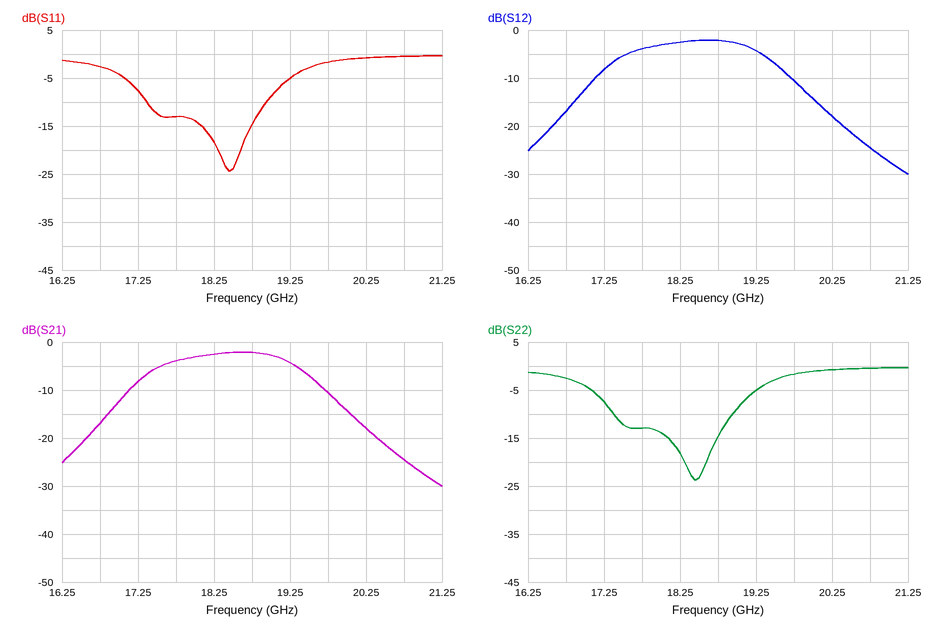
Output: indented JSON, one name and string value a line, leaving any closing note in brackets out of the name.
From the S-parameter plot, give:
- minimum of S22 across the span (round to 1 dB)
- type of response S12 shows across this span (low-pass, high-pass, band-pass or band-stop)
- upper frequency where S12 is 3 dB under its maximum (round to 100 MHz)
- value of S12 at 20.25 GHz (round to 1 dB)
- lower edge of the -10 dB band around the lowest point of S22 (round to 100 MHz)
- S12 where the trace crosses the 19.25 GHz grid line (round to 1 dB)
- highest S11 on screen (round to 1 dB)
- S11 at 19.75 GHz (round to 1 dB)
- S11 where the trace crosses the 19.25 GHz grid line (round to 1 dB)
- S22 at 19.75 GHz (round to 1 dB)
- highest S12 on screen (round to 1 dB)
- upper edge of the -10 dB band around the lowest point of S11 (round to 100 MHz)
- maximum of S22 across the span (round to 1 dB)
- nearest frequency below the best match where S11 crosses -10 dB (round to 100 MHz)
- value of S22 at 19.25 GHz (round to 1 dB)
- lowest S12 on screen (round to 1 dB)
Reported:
{
  "minimum of S22 across the span": "-24 dB",
  "type of response S12 shows across this span": "band-pass",
  "upper frequency where S12 is 3 dB under its maximum": "19.3 GHz",
  "value of S12 at 20.25 GHz": "-18 dB",
  "lower edge of the -10 dB band around the lowest point of S22": "17.4 GHz",
  "S12 where the trace crosses the 19.25 GHz grid line": "-4 dB",
  "highest S11 on screen": "0 dB",
  "S11 at 19.75 GHz": "-2 dB",
  "S11 where the trace crosses the 19.25 GHz grid line": "-5 dB",
  "S22 at 19.75 GHz": "-2 dB",
  "highest S12 on screen": "-2 dB",
  "upper edge of the -10 dB band around the lowest point of S11": "18.9 GHz",
  "maximum of S22 across the span": "0 dB",
  "nearest frequency below the best match where S11 crosses -10 dB": "17.4 GHz",
  "value of S22 at 19.25 GHz": "-5 dB",
  "lowest S12 on screen": "-30 dB"
}
